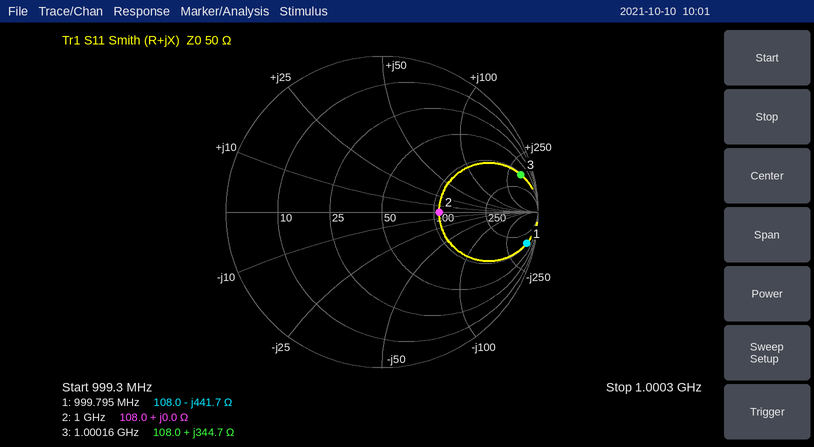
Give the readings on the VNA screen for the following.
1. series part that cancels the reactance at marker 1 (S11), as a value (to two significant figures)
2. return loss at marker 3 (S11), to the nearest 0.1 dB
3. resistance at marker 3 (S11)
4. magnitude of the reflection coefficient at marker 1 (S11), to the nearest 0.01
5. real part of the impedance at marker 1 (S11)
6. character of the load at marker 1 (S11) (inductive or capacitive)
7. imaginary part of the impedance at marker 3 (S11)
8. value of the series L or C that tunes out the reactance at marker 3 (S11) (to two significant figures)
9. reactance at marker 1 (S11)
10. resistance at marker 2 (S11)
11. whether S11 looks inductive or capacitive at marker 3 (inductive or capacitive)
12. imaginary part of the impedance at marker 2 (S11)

70 nH
0.7 dB
108.0 Ω
0.95
108.0 Ω
capacitive
+344.7 Ω
460 fF
-441.7 Ω
108.0 Ω
inductive
+0.0 Ω
